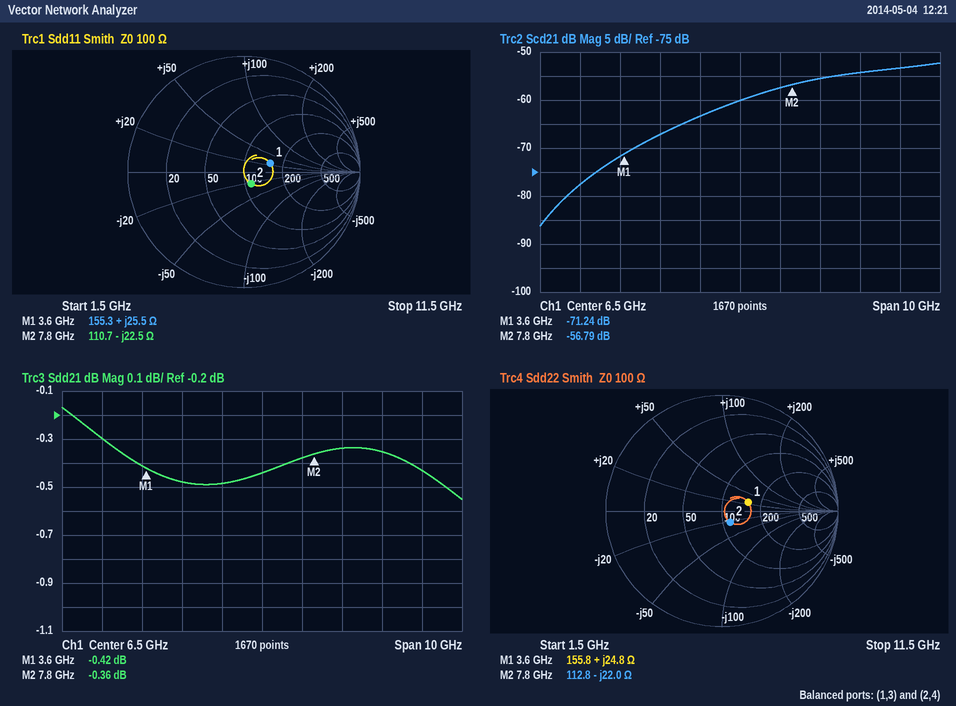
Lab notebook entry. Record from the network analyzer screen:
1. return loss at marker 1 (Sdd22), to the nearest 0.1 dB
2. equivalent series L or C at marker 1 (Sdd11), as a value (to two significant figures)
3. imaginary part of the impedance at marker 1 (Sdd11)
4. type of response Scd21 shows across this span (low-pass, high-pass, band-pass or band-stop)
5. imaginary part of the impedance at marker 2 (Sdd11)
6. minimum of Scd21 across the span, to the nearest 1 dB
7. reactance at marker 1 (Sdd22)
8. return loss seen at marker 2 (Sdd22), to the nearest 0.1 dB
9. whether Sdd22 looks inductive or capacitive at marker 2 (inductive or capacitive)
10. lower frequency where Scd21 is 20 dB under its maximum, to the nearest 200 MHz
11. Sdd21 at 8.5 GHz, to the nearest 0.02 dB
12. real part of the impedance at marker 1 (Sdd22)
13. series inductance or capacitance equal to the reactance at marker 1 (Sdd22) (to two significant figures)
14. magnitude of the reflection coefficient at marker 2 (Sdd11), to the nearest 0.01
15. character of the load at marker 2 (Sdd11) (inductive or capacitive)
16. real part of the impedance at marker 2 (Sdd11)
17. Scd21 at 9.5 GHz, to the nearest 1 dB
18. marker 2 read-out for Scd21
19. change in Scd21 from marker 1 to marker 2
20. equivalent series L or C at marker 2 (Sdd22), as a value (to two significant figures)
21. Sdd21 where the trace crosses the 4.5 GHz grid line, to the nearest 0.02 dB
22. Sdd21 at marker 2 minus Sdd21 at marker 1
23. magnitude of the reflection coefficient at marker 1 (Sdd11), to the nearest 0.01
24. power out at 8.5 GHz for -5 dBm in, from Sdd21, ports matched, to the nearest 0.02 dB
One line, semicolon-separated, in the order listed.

12.5 dB; 1.1 nH; +25.5 Ω; high-pass; -22.5 Ω; -86 dB; +24.8 Ω; 18.5 dB; capacitive; 3.4 GHz; -0.34 dB; 155.8 Ω; 1.1 nH; 0.12; capacitive; 110.7 Ω; -54 dB; -56.79 dB; 14.45 dB; 930 fF; -0.48 dB; 0.06 dB; 0.24; -5.34 dBm
